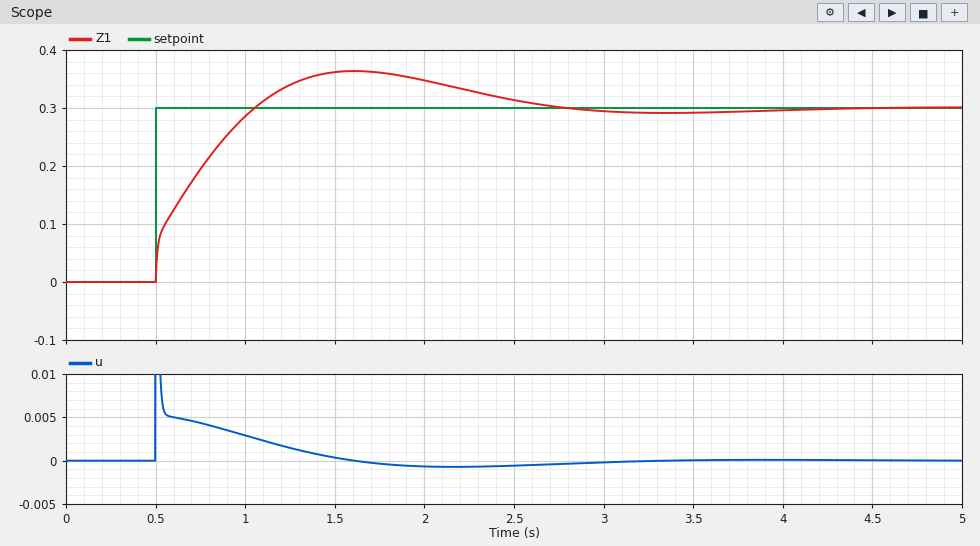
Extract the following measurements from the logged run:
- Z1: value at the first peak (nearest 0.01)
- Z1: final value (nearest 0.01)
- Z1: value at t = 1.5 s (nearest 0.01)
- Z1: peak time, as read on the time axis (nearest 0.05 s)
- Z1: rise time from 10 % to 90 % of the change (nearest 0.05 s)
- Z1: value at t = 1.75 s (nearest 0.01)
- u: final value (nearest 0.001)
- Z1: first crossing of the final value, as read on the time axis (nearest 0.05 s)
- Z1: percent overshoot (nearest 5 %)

0.36
0.30
0.36
1.60 s
0.45 s
0.36
0.000
1.05 s
20 %
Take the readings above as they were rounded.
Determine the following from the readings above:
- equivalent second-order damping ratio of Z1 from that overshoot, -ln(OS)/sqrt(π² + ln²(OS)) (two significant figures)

0.46
